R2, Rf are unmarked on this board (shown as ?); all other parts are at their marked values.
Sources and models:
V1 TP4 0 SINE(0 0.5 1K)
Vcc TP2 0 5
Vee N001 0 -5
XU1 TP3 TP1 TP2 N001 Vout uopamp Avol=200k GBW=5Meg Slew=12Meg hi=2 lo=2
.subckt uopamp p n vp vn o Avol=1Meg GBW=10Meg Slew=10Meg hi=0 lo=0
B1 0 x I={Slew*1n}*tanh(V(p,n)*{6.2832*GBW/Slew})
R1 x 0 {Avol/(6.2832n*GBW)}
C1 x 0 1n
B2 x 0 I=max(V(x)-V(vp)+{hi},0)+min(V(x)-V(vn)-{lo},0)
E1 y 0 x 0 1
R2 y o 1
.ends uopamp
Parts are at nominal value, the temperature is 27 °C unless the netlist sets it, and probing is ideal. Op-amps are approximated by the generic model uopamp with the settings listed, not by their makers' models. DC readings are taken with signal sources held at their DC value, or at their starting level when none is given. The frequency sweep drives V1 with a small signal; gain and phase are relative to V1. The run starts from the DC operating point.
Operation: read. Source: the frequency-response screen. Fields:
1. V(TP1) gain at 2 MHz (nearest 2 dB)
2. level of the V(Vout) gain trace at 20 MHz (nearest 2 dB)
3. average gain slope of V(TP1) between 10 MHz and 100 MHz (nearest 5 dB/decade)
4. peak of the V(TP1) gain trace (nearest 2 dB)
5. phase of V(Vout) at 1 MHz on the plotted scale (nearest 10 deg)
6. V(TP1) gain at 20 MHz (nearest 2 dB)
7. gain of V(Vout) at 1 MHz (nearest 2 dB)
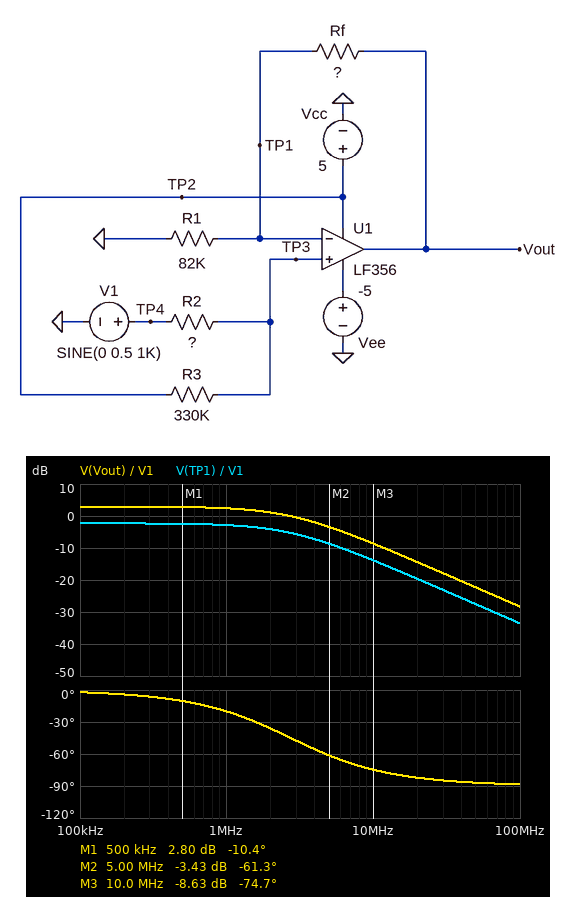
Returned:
-4 dB
-14 dB
-20 dB/decade
-2 dB
-20 deg
-20 dB
2 dB
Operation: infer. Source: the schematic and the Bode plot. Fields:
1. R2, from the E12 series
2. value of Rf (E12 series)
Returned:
100 kΩ
68 kΩ
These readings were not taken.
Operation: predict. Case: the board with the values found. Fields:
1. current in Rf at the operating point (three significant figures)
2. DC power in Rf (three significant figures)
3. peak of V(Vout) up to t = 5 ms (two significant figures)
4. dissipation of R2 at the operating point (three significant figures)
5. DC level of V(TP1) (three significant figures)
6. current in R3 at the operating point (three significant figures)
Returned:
14.2 µA
13.7 µW
2.8 V
13.5 µW
1.16 V
11.6 µA
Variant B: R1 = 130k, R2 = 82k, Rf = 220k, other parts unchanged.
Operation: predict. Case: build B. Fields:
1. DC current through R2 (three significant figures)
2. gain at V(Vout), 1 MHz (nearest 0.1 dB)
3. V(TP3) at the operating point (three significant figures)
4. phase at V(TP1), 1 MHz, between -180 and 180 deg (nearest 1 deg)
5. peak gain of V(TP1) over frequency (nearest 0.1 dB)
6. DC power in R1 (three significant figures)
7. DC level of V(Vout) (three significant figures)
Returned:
12.1 µA
5.6 dB
995 mV
-28 deg
-1.9 dB
7.62 µW
2.68 V
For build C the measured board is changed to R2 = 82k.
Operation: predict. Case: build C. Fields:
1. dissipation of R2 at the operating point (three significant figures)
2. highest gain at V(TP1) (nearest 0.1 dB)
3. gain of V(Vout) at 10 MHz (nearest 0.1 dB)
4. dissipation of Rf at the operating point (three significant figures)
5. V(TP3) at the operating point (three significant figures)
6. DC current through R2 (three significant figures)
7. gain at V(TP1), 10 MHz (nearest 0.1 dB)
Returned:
12.1 µW
-1.9 dB
-8.3 dB
10.0 µW
995 mV
12.1 µA
-13.5 dB
